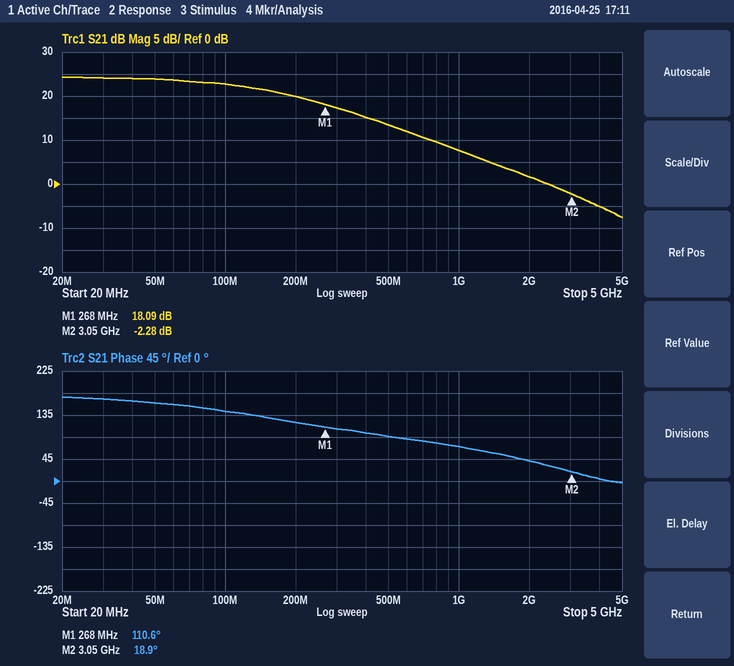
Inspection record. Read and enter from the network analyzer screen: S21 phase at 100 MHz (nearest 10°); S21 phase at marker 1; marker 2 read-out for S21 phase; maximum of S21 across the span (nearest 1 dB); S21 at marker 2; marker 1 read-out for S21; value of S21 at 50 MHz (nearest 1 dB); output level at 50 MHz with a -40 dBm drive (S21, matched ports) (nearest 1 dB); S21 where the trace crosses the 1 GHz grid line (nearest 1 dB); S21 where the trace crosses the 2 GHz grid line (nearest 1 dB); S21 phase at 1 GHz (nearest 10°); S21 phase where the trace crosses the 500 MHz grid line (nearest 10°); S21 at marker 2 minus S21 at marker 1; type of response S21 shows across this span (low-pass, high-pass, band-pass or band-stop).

140°
110.6°
18.9°
24 dB
-2.28 dB
18.09 dB
24 dB
-16 dBm
8 dB
2 dB
70°
90°
-20.37 dB
low-pass
